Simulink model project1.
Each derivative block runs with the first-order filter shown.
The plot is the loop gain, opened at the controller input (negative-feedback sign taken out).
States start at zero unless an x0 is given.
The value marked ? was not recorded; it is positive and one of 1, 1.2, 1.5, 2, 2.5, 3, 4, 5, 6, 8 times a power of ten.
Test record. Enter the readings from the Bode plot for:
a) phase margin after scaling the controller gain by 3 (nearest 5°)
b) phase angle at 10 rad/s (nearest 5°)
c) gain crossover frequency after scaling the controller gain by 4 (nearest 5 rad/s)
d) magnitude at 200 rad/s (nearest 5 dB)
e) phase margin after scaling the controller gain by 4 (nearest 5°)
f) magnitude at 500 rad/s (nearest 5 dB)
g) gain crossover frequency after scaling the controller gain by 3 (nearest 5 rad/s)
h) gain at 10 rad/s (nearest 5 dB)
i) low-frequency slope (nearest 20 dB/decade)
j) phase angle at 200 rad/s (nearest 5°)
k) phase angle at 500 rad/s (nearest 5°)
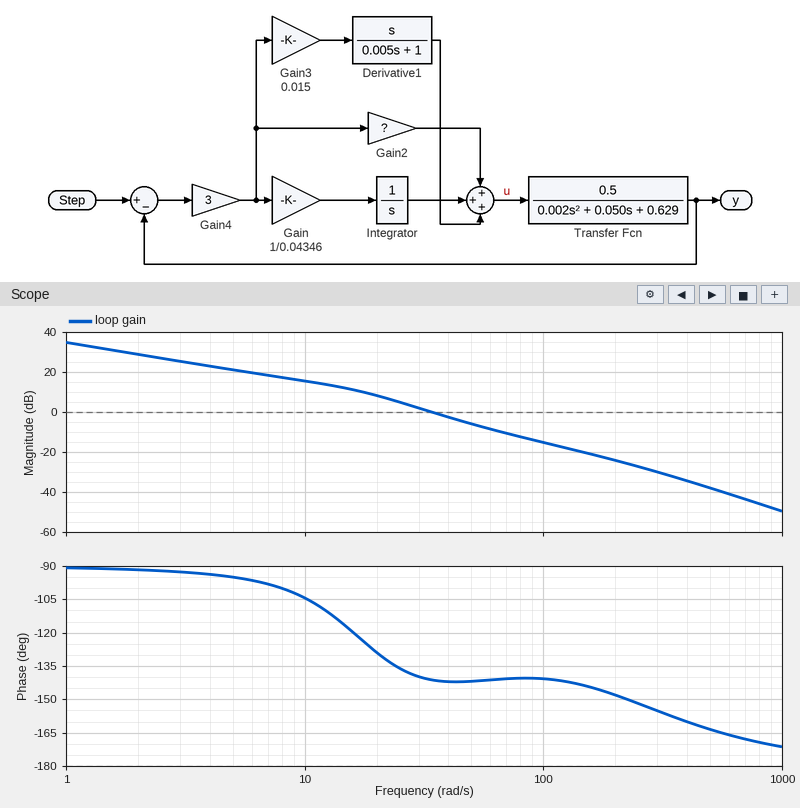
40°
-105°
80 rad/s
-25 dB
40°
-40 dB
65 rad/s
15 dB
-20 dB/decade
-150°
-165°
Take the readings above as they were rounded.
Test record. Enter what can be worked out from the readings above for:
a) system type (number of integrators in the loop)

1
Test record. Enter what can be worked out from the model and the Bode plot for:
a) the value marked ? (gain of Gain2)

1.5
